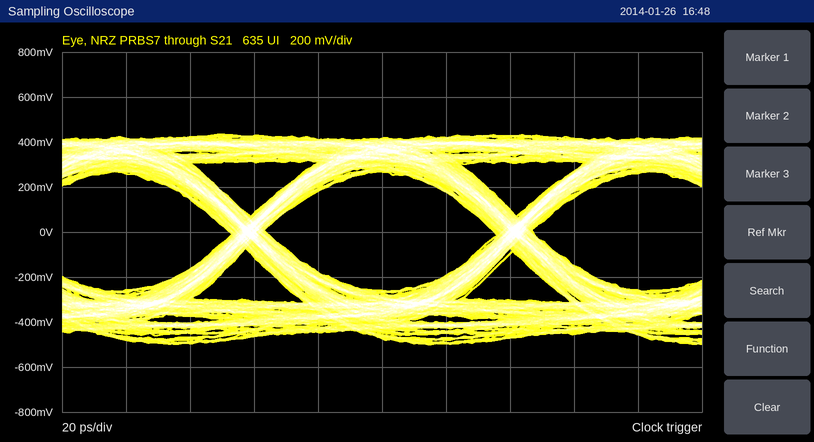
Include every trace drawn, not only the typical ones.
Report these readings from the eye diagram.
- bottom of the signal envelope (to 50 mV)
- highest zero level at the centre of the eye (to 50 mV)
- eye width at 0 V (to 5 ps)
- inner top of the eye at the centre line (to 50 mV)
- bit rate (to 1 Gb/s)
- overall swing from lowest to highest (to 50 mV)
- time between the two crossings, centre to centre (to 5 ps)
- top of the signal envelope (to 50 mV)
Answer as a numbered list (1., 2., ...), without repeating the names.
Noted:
1. -500 mV
2. -250 mV
3. 70 ps
4. 250 mV
5. 12 Gb/s
6. 950 mV
7. 85 ps
8. 450 mV
